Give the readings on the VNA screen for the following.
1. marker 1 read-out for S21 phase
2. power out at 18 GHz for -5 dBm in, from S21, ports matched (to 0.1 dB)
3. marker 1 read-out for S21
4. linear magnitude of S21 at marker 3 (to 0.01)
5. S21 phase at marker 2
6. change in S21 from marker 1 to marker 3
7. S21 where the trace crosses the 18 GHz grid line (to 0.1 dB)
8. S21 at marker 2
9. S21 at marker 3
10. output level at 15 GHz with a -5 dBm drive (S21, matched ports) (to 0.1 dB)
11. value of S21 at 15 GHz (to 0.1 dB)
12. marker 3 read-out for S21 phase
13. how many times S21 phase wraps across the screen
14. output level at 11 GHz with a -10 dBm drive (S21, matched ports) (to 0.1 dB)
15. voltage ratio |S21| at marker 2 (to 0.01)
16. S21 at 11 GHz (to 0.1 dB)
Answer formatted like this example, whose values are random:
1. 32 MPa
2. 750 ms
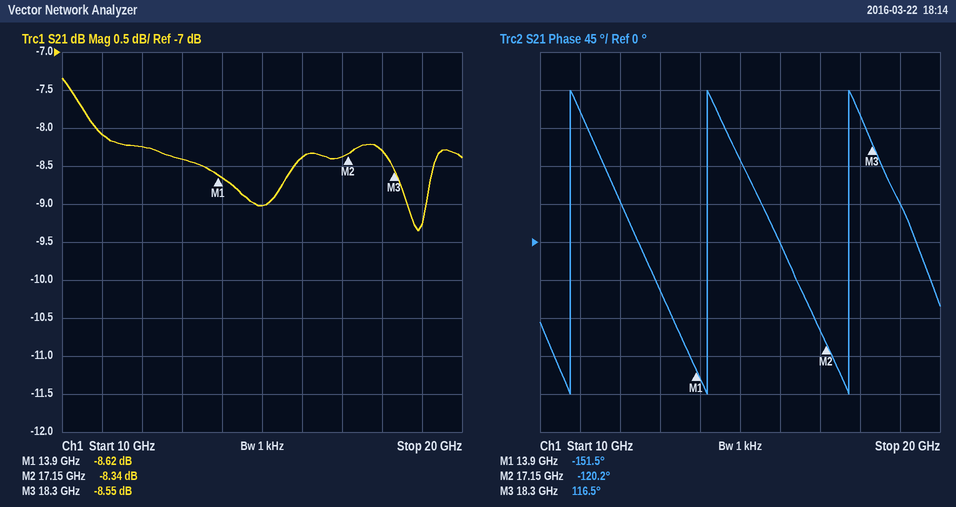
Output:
1. -151.5°
2. -13.3 dBm
3. -8.62 dB
4. 0.37
5. -120.2°
6. 0.07 dB
7. -8.3 dB
8. -8.34 dB
9. -8.55 dB
10. -14.0 dBm
11. -9.0 dB
12. 116.5°
13. 3
14. -18.1 dBm
15. 0.38
16. -8.1 dB
